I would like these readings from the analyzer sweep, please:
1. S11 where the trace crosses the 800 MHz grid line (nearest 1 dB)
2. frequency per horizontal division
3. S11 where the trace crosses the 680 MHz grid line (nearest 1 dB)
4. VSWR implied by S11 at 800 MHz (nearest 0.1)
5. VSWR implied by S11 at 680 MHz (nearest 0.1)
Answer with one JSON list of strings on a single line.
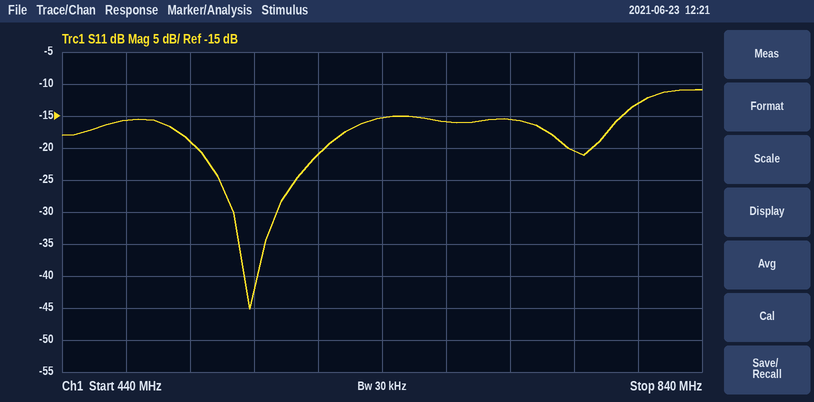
["-13 dB", "40 MHz", "-16 dB", "1.6", "1.4"]
